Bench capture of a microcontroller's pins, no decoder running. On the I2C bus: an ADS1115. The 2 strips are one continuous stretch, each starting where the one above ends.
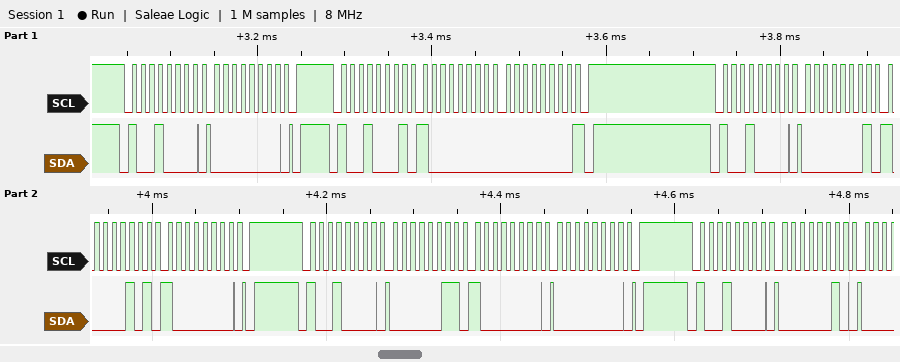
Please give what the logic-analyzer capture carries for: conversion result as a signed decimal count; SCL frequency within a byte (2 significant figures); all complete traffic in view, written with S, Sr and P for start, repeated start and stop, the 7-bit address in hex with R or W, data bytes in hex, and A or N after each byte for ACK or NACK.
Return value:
-32768
100 kHz
S 48W A 00 A P S 48R A 80 A 00 N P S 48W A 01 A 85 A 80 A P S 48W A 03 A 80 A 00 A P S 48W A 02 A
